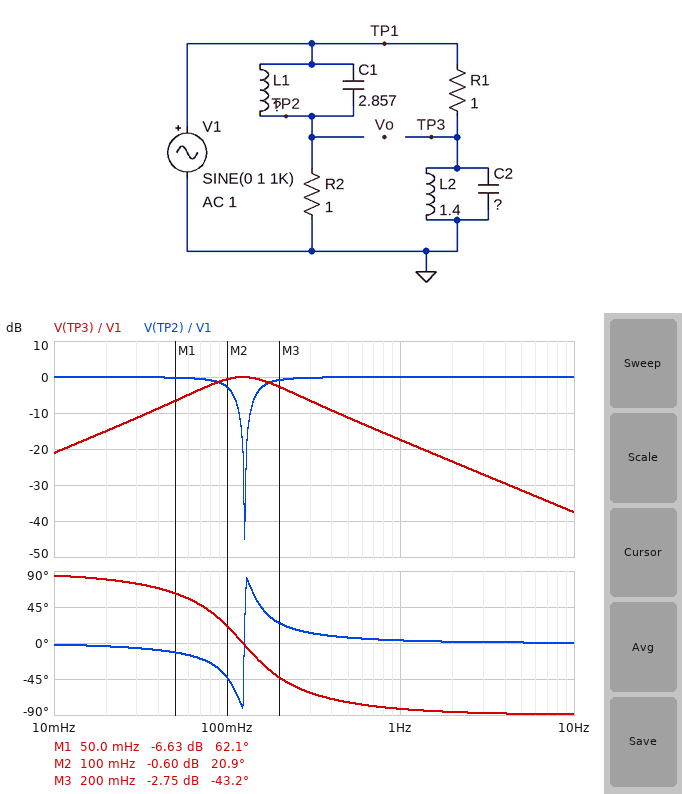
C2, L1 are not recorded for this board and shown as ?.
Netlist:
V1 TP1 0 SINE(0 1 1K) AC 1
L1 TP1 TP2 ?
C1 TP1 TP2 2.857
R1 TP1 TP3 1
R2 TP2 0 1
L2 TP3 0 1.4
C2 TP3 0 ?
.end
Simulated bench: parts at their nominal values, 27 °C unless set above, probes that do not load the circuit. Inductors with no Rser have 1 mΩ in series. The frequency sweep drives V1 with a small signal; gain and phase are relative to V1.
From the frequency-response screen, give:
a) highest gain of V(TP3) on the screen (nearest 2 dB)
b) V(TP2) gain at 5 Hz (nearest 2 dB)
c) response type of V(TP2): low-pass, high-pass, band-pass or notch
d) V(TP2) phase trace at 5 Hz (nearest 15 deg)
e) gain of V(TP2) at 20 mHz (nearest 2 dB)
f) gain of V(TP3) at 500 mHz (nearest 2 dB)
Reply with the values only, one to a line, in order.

0 dB
0 dB
notch
0 deg
0 dB
-12 dB
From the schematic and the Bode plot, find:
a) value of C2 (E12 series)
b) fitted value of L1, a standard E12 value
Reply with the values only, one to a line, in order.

1.2 F
560 mH
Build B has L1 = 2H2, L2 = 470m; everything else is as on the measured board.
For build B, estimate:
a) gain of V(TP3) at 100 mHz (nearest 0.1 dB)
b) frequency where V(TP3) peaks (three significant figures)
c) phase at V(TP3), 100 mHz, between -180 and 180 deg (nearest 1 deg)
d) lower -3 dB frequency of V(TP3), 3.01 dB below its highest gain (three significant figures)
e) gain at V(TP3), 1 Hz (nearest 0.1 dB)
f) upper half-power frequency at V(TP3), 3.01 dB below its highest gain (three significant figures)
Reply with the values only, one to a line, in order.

-9.0 dB
212 mHz
69 deg
156 mHz
-17.2 dB
289 mHz
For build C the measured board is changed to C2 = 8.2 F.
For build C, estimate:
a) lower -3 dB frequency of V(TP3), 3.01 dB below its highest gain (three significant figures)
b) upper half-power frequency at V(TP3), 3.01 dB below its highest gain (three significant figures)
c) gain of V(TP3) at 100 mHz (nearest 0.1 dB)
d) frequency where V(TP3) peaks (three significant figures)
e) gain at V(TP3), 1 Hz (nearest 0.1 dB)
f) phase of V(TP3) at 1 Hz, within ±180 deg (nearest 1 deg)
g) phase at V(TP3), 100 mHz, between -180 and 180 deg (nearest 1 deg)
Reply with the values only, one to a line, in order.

38.2 mHz
57.8 mHz
-12.3 dB
47.0 mHz
-34.2 dB
-89 deg
-76 deg
